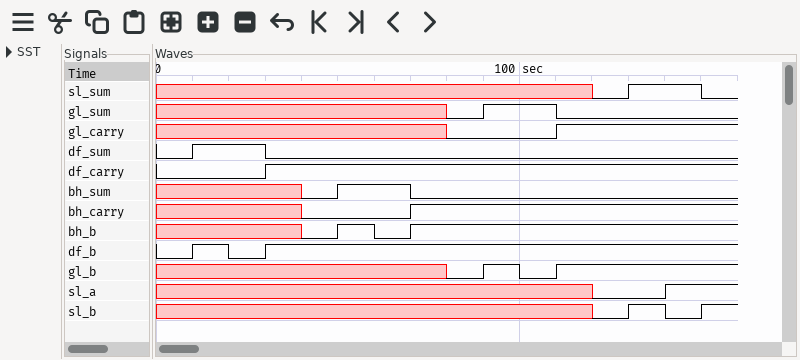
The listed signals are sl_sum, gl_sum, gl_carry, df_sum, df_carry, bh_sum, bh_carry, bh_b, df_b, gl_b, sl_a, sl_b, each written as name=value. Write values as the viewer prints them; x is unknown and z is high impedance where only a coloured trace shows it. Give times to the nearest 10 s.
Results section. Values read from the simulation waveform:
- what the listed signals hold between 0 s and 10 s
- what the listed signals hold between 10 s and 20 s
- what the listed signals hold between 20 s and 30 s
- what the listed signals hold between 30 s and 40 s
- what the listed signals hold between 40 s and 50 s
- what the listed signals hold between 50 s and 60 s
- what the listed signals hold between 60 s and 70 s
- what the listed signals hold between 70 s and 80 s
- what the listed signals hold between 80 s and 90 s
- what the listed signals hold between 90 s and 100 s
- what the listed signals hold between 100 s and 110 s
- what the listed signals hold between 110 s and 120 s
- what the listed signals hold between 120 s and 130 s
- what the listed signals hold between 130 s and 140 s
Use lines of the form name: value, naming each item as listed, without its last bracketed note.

what the listed signals hold between 0 s and 10 s: sl_sum=x, gl_sum=x, gl_carry=x, df_sum=0, df_carry=0, bh_sum=x, bh_carry=x, bh_b=x, df_b=0, gl_b=x, sl_a=x, sl_b=x
what the listed signals hold between 10 s and 20 s: sl_sum=x, gl_sum=x, gl_carry=x, df_sum=1, df_carry=0, bh_sum=x, bh_carry=x, bh_b=x, df_b=1, gl_b=x, sl_a=x, sl_b=x
what the listed signals hold between 20 s and 30 s: sl_sum=x, gl_sum=x, gl_carry=x, df_sum=1, df_carry=0, bh_sum=x, bh_carry=x, bh_b=x, df_b=0, gl_b=x, sl_a=x, sl_b=x
what the listed signals hold between 30 s and 40 s: sl_sum=x, gl_sum=x, gl_carry=x, df_sum=0, df_carry=1, bh_sum=x, bh_carry=x, bh_b=x, df_b=1, gl_b=x, sl_a=x, sl_b=x
what the listed signals hold between 40 s and 50 s: sl_sum=x, gl_sum=x, gl_carry=x, df_sum=0, df_carry=1, bh_sum=0, bh_carry=0, bh_b=0, df_b=1, gl_b=x, sl_a=x, sl_b=x
what the listed signals hold between 50 s and 60 s: sl_sum=x, gl_sum=x, gl_carry=x, df_sum=0, df_carry=1, bh_sum=1, bh_carry=0, bh_b=1, df_b=1, gl_b=x, sl_a=x, sl_b=x
what the listed signals hold between 60 s and 70 s: sl_sum=x, gl_sum=x, gl_carry=x, df_sum=0, df_carry=1, bh_sum=1, bh_carry=0, bh_b=0, df_b=1, gl_b=x, sl_a=x, sl_b=x
what the listed signals hold between 70 s and 80 s: sl_sum=x, gl_sum=x, gl_carry=x, df_sum=0, df_carry=1, bh_sum=0, bh_carry=1, bh_b=1, df_b=1, gl_b=x, sl_a=x, sl_b=x
what the listed signals hold between 80 s and 90 s: sl_sum=x, gl_sum=0, gl_carry=0, df_sum=0, df_carry=1, bh_sum=0, bh_carry=1, bh_b=1, df_b=1, gl_b=0, sl_a=x, sl_b=x
what the listed signals hold between 90 s and 100 s: sl_sum=x, gl_sum=1, gl_carry=0, df_sum=0, df_carry=1, bh_sum=0, bh_carry=1, bh_b=1, df_b=1, gl_b=1, sl_a=x, sl_b=x
what the listed signals hold between 100 s and 110 s: sl_sum=x, gl_sum=1, gl_carry=0, df_sum=0, df_carry=1, bh_sum=0, bh_carry=1, bh_b=1, df_b=1, gl_b=0, sl_a=x, sl_b=x
what the listed signals hold between 110 s and 120 s: sl_sum=x, gl_sum=0, gl_carry=1, df_sum=0, df_carry=1, bh_sum=0, bh_carry=1, bh_b=1, df_b=1, gl_b=1, sl_a=x, sl_b=x
what the listed signals hold between 120 s and 130 s: sl_sum=0, gl_sum=0, gl_carry=1, df_sum=0, df_carry=1, bh_sum=0, bh_carry=1, bh_b=1, df_b=1, gl_b=1, sl_a=0, sl_b=0
what the listed signals hold between 130 s and 140 s: sl_sum=1, gl_sum=0, gl_carry=1, df_sum=0, df_carry=1, bh_sum=0, bh_carry=1, bh_b=1, df_b=1, gl_b=1, sl_a=0, sl_b=1
